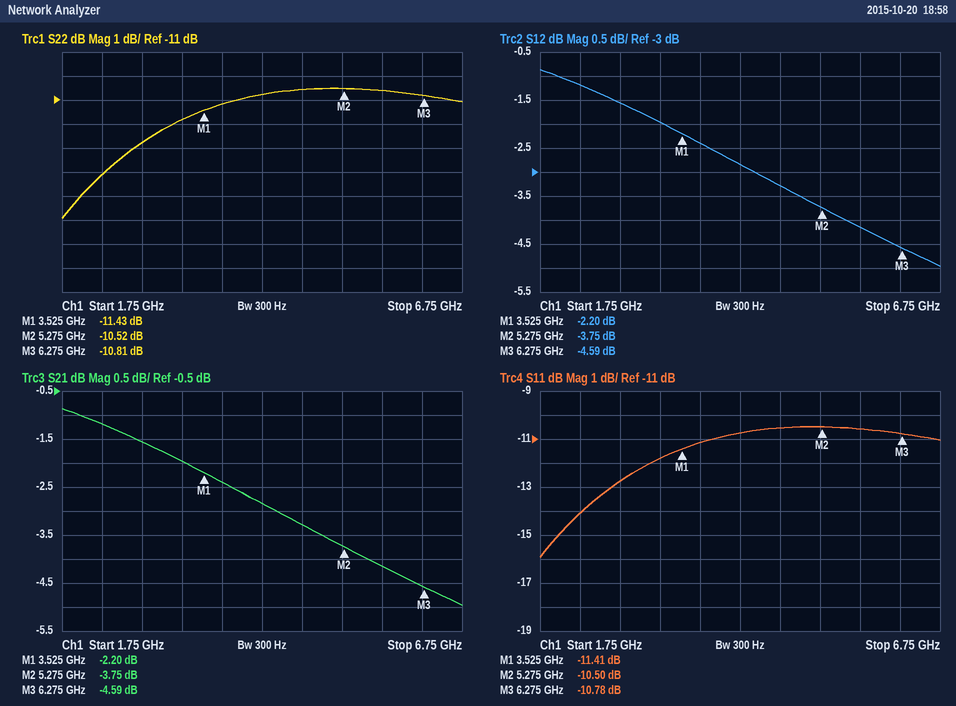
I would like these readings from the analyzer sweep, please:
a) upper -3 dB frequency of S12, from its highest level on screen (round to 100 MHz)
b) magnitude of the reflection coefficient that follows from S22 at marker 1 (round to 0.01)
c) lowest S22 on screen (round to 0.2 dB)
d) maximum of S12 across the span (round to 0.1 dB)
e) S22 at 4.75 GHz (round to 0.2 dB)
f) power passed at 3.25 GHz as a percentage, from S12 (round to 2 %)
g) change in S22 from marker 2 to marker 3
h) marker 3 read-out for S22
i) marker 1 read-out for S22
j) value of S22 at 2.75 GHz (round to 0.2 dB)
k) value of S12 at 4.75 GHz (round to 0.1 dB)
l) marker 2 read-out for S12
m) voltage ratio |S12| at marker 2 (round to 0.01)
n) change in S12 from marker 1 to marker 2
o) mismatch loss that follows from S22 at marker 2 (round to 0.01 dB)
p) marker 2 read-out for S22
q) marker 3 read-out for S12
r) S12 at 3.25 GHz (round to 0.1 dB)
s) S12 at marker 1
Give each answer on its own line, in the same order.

5.4 GHz
0.27
-16.0 dB
-0.9 dB
-10.6 dB
64 %
-0.29 dB
-10.81 dB
-11.43 dB
-12.8 dB
-3.3 dB
-3.75 dB
0.65
-1.55 dB
0.40 dB
-10.52 dB
-4.59 dB
-2.0 dB
-2.20 dB
